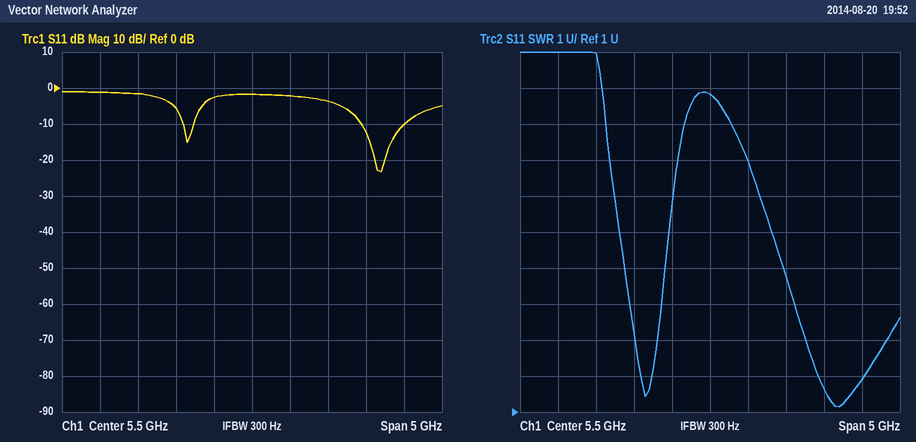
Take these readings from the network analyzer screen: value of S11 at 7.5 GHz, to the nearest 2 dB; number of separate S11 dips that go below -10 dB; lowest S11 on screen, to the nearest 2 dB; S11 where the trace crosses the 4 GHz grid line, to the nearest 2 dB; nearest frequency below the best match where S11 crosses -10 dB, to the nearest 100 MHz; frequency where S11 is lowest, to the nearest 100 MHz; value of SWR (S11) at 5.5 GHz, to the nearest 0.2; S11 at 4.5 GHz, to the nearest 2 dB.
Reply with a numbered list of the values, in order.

1. -10 dB
2. 2
3. -24 dB
4. -2 dB
5. 6.9 GHz
6. 7.2 GHz
7. 9.8
8. -6 dB
